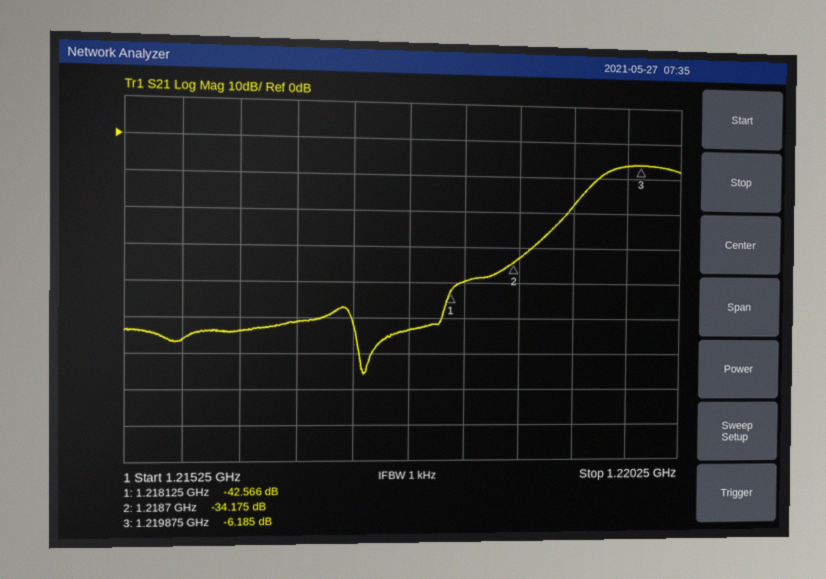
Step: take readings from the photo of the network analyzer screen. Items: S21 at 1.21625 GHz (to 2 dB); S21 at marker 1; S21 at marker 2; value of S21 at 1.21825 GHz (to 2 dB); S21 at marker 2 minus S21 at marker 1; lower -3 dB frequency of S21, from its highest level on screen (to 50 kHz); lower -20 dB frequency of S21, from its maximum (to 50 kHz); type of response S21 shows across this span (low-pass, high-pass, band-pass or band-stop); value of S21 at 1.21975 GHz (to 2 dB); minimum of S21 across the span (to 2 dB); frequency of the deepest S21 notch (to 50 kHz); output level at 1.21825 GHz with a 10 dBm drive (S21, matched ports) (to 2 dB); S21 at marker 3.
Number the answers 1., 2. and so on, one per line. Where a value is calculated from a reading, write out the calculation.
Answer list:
1. -54 dB
2. -42.566 dB
3. -34.175 dB
4. -40 dB
5. -34.175 − (-42.566) = 8.391 dB
6. 1.21950 GHz
7. 1.21900 GHz
8. high-pass
9. -6 dB
10. -66 dB
11. 1.21735 GHz
12. 10 dBm + (-40 dB) = -30 dBm
13. -6.185 dB
